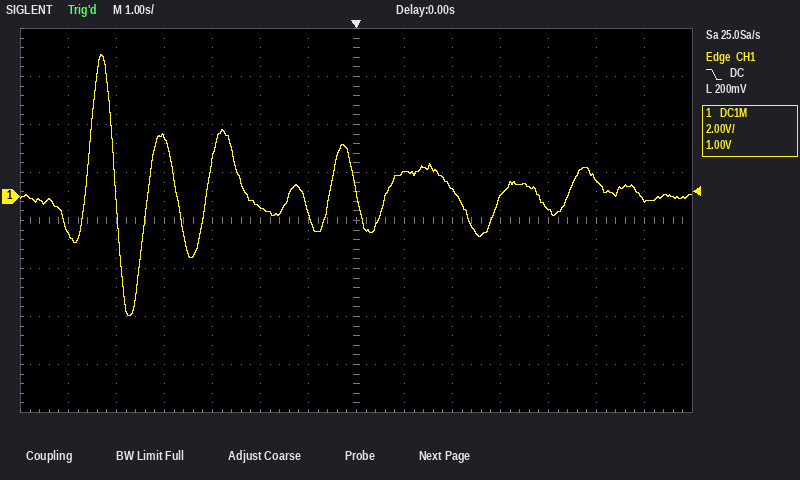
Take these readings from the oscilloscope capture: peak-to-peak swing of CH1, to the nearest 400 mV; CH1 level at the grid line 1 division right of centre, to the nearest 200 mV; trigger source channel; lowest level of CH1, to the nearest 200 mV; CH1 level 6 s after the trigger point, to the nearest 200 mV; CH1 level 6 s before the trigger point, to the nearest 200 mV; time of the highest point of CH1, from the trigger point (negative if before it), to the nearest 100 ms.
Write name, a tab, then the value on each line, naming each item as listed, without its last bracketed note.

peak-to-peak swing of CH1, to the nearest 400 mV	10.8 V
CH1 level at the grid line 1 division right of centre, to the nearest 200 mV	1.0 V
trigger source channel	CH1
lowest level of CH1, to the nearest 200 mV	-5.0 V
CH1 level 6 s after the trigger point, to the nearest 200 mV	-200 mV
CH1 level 6 s before the trigger point, to the nearest 200 mV	-1.6 V
time of the highest point of CH1, from the trigger point (negative if before it), to the nearest 100 ms	-5.3 s
